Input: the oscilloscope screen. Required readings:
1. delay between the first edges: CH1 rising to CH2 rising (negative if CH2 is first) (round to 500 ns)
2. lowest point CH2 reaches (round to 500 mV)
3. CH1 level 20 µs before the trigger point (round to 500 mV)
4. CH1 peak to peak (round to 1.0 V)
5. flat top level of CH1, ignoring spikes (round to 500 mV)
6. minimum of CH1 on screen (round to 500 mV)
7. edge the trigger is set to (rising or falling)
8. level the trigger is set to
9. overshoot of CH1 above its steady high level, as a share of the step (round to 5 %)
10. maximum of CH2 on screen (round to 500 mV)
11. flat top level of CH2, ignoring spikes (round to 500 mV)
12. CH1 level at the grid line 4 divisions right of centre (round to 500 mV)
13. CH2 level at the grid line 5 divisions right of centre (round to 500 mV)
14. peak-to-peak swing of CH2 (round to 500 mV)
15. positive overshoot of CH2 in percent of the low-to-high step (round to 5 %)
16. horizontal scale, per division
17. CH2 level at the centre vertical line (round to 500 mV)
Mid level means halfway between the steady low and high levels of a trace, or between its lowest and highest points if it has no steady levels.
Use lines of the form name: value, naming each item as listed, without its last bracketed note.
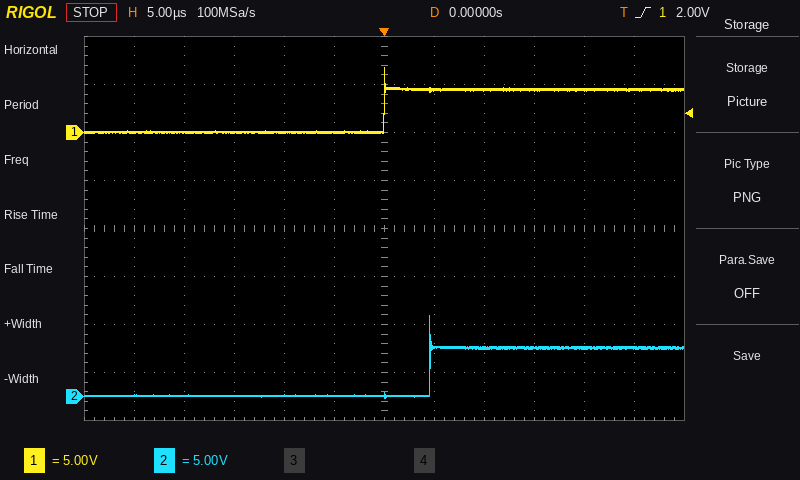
delay between the first edges: CH1 rising to CH2 rising (negative if CH2 is first): +4.5 µs
lowest point CH2 reaches: 0.0 V
CH1 level 20 µs before the trigger point: 0.0 V
CH1 peak to peak: 7.0 V
flat top level of CH1, ignoring spikes: 4.5 V
minimum of CH1 on screen: 0.0 V
edge the trigger is set to: rising
level the trigger is set to: 2.00 V
overshoot of CH1 above its steady high level, as a share of the step: 50 %
maximum of CH2 on screen: 8.5 V
flat top level of CH2, ignoring spikes: 5.0 V
CH1 level at the grid line 4 divisions right of centre: 4.5 V
CH2 level at the grid line 5 divisions right of centre: 5.0 V
peak-to-peak swing of CH2: 8.5 V
positive overshoot of CH2 in percent of the low-to-high step: 65 %
horizontal scale, per division: 5 µs
CH2 level at the centre vertical line: 0.0 V
